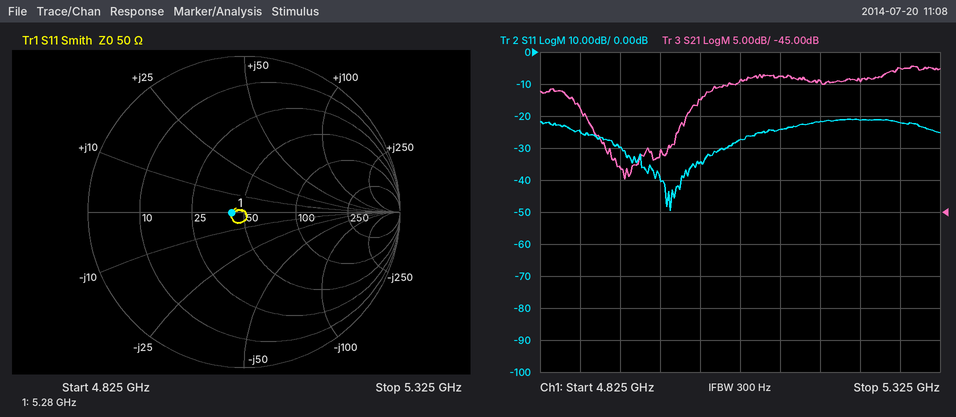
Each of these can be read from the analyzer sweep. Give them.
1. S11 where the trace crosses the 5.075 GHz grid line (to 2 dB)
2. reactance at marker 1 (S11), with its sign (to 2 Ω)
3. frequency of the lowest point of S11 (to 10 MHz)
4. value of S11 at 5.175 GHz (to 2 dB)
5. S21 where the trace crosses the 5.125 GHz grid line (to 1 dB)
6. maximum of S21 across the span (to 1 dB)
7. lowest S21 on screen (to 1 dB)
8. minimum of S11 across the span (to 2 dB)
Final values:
-28 dB
0 Ω
4.99 GHz
-22 dB
-24 dB
-22 dB
-40 dB
-50 dB
